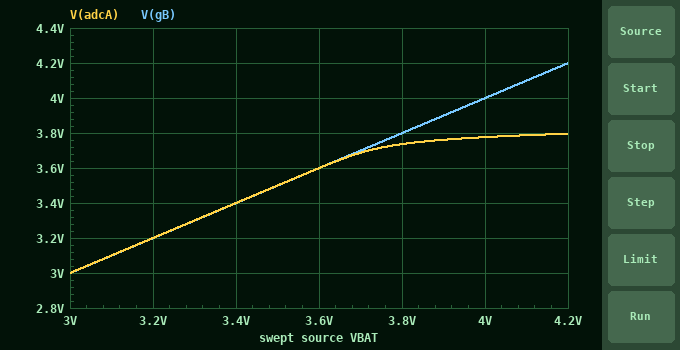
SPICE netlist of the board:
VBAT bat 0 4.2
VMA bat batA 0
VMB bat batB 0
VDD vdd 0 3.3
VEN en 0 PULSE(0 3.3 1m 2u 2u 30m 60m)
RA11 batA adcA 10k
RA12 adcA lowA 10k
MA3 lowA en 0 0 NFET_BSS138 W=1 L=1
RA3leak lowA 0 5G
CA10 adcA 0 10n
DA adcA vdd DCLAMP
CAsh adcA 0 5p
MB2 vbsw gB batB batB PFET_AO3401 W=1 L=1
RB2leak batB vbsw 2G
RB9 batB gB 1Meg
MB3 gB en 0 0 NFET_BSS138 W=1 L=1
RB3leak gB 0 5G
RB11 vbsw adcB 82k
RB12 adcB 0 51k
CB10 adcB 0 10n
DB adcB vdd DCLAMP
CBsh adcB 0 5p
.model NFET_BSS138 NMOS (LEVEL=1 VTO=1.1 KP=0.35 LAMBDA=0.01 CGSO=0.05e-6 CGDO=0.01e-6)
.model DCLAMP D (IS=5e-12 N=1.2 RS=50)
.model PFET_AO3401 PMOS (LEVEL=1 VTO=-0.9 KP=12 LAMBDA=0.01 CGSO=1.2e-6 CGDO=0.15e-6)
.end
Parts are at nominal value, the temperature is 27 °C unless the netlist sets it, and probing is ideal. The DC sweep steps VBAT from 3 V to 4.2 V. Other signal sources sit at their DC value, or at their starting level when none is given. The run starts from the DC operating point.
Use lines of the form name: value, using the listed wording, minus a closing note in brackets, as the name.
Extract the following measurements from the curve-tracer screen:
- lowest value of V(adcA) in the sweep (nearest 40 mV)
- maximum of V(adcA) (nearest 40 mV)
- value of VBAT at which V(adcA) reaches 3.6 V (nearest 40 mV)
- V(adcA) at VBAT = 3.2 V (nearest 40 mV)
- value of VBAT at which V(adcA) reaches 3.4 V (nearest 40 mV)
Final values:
lowest value of V(adcA) in the sweep: 3.00 V
maximum of V(adcA): 3.80 V
value of VBAT at which V(adcA) reaches 3.6 V: 3.60 V
V(adcA) at VBAT = 3.2 V: 3.20 V
value of VBAT at which V(adcA) reaches 3.4 V: 3.40 V
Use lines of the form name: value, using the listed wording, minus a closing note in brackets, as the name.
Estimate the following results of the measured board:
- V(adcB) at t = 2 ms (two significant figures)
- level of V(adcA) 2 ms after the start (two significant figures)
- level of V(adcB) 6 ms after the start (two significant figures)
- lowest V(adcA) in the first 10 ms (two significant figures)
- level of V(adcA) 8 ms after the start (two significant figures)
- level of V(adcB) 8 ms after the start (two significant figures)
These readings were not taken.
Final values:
V(adcB) at t = 2 ms: 1.5 V
level of V(adcA) 2 ms after the start: 2.1 V
level of V(adcB) 6 ms after the start: 1.6 V
lowest V(adcA) in the first 10 ms: 2.1 V
level of V(adcA) 8 ms after the start: 2.1 V
level of V(adcB) 8 ms after the start: 1.6 V
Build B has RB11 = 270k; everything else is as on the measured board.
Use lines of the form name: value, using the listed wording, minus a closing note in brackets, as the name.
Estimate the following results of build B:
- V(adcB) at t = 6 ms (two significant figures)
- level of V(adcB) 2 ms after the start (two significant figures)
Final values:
V(adcB) at t = 6 ms: 670 mV
level of V(adcB) 2 ms after the start: 600 mV
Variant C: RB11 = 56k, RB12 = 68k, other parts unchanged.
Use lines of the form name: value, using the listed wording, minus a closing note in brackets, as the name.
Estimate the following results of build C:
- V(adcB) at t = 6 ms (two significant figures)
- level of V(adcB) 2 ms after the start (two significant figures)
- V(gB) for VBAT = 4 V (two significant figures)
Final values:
V(adcB) at t = 6 ms: 2.3 V
level of V(adcB) 2 ms after the start: 2.2 V
V(gB) for VBAT = 4 V: 4.0 V
